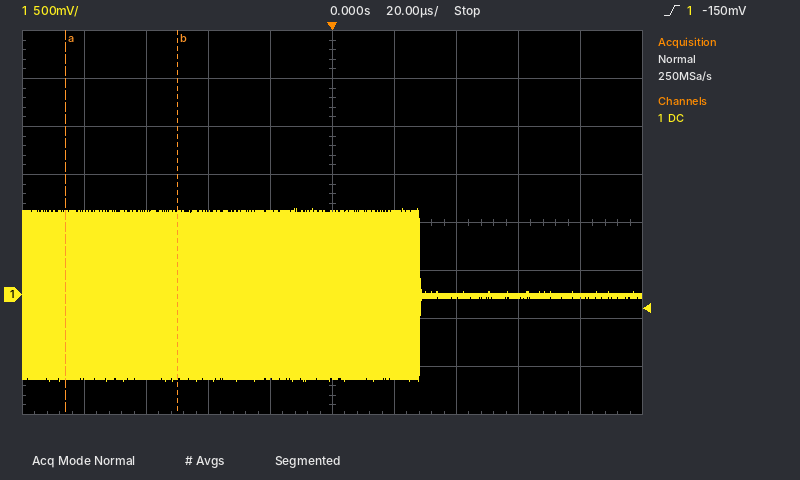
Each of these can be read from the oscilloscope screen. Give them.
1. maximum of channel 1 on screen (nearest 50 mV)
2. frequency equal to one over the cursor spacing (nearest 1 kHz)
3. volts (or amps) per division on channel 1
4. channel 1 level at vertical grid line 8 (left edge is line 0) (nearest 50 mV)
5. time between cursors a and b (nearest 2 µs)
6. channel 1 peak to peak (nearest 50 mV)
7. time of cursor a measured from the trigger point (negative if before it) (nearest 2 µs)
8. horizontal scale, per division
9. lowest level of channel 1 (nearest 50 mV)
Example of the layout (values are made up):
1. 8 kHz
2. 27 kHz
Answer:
1. 900 mV
2. 28 kHz
3. 500 mV
4. 0 mV
5. 36 µs
6. 1.80 V
7. -86 µs
8. 20 µs
9. -900 mV
